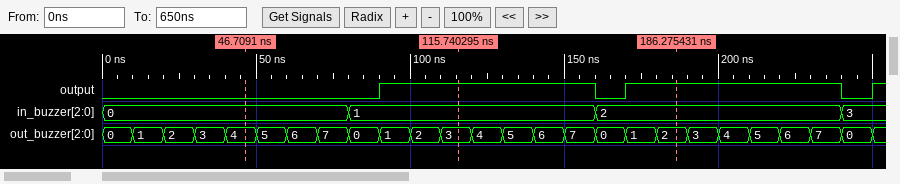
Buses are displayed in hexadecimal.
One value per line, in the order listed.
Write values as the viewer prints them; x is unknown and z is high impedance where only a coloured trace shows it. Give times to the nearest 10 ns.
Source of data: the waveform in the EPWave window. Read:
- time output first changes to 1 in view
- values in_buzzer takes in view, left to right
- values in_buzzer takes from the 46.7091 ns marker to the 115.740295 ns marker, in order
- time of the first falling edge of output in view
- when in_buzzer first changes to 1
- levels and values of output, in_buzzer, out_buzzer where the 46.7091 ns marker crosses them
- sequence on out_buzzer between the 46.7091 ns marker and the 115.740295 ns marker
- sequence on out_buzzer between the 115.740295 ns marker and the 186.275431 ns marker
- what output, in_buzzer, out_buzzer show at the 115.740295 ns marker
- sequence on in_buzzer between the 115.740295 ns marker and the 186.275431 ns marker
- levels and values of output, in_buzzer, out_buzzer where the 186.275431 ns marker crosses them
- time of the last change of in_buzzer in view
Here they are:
90 ns
0, 1, 2, 3
0, 1
160 ns
80 ns
output=0, in_buzzer=0, out_buzzer=4
4, 5, 6, 7, 0, 1, 2, 3
3, 4, 5, 6, 7, 0, 1, 2
output=1, in_buzzer=1, out_buzzer=3
1, 2
output=1, in_buzzer=2, out_buzzer=2
240 ns
